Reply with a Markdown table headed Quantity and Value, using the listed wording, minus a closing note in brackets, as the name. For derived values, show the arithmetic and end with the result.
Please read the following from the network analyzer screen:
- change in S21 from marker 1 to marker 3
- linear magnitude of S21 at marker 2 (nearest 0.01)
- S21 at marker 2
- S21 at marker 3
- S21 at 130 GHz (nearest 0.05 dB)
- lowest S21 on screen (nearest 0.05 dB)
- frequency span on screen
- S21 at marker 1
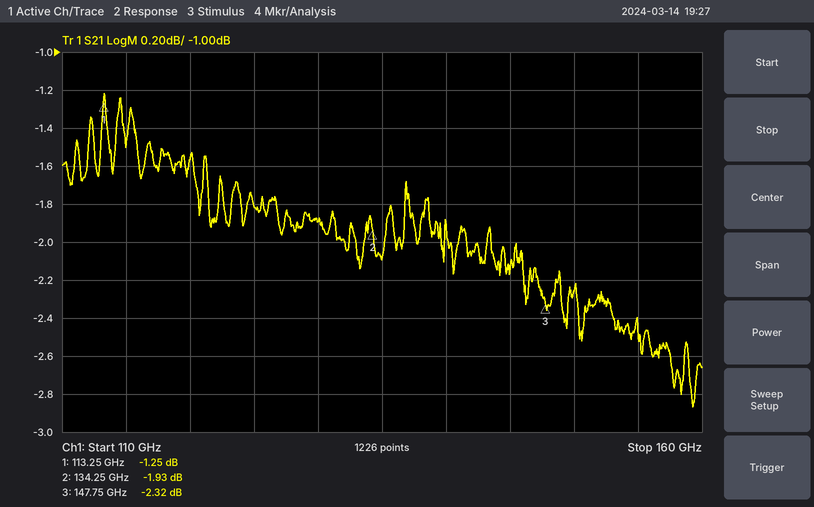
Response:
| Quantity | Value |
|---|---|
| change in S21 from marker 1 to marker 3 | -2.32 − (-1.25) = -1.07 dB |
| linear magnitude of S21 at marker 2 | 10^(-1.93/20) ≈ 0.80 |
| S21 at marker 2 | -1.93 dB |
| S21 at marker 3 | -2.32 dB |
| S21 at 130 GHz | -1.90 dB |
| lowest S21 on screen | -2.85 dB |
| frequency span on screen | 50 GHz |
| S21 at marker 1 | -1.25 dB |
